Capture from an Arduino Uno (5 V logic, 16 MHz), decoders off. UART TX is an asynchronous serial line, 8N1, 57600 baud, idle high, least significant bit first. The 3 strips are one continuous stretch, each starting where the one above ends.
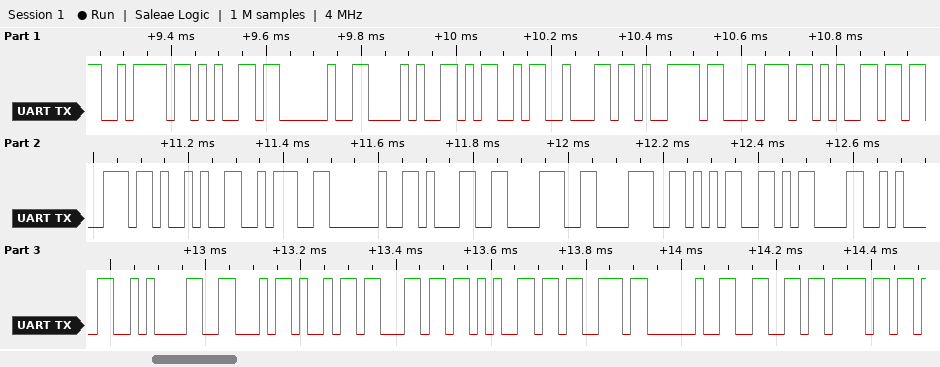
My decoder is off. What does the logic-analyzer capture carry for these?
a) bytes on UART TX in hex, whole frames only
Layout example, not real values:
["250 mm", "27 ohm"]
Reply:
["0x7A 0x65 0x20 0x28 0x4D 0x62 0x79 0x74 0x65 0x73 0x29 0x3A 0x20 0x31 0x38 0x38 0x35 0x0D 0x0A 0x0A 0x46 0x69 0x6C 0x65 0x73 0x20 0x66 0x6F"]
